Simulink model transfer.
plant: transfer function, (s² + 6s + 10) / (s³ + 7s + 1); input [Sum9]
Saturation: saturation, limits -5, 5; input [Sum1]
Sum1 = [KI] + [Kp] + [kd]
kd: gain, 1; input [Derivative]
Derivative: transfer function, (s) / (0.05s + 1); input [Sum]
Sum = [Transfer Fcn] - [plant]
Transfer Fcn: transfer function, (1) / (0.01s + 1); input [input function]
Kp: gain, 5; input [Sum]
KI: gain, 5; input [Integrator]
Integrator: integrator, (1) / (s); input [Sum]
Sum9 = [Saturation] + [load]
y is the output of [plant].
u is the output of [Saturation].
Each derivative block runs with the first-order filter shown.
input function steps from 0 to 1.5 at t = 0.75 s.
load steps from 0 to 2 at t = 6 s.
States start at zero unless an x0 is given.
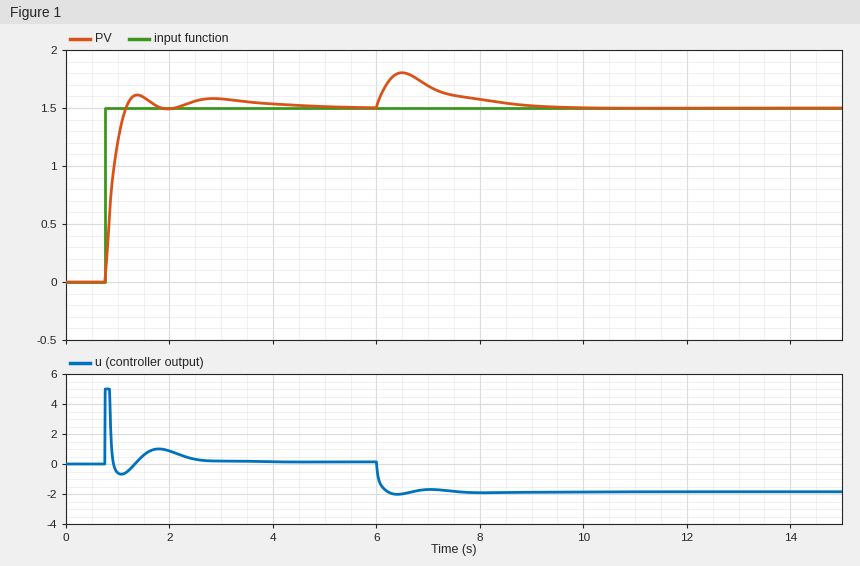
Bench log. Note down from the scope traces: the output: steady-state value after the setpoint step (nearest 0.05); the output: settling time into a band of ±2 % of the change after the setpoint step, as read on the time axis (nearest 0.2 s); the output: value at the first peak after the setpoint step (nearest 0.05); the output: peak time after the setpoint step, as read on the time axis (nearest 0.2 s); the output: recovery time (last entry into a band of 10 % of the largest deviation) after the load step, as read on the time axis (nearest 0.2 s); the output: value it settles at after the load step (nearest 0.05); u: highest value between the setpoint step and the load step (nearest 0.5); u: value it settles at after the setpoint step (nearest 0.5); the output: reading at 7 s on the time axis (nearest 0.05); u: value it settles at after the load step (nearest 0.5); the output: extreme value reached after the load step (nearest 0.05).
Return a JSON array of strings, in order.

["1.50", "4.2 s", "1.60", "1.4 s", "8.8 s", "1.50", "5.0", "0.0", "1.70", "-2.0", "1.80"]
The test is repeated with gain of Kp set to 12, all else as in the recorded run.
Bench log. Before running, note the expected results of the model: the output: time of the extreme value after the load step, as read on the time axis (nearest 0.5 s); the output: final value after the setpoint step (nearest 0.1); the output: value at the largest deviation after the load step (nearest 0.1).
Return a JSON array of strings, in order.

["6.5 s", "1.5", "1.7"]
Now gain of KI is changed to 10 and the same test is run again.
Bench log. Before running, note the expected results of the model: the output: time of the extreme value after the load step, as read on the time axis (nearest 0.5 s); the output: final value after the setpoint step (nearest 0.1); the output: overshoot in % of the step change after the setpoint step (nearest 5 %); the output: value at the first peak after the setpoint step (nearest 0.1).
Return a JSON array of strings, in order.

["6.5 s", "1.5", "15 %", "1.7"]
